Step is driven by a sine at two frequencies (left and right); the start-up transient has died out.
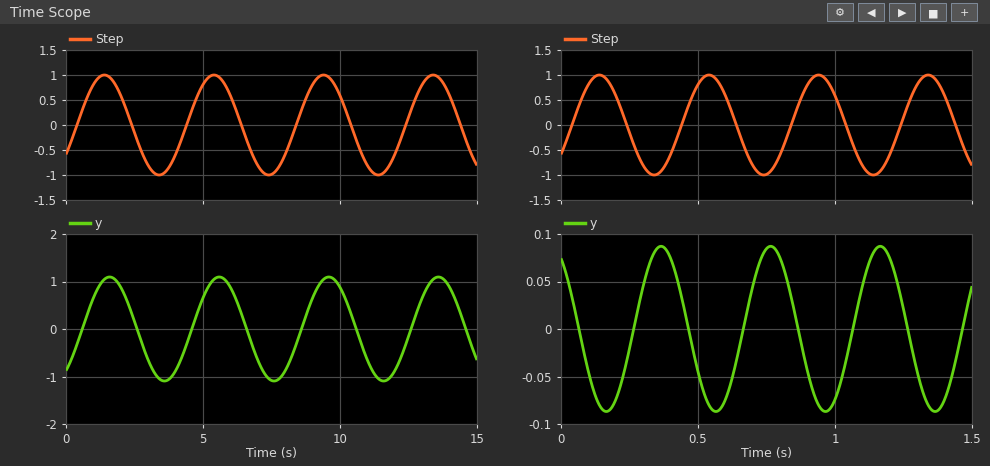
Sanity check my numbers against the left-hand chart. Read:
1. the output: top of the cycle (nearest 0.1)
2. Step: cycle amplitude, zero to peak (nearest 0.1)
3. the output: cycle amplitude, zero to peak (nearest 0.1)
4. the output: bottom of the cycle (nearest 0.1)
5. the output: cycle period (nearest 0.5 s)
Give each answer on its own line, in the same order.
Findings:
1.1
1.0
1.1
-1.1
4.0 s
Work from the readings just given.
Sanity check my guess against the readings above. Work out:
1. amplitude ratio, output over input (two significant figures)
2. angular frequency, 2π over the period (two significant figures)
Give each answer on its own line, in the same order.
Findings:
1.1
1.6 rad/s
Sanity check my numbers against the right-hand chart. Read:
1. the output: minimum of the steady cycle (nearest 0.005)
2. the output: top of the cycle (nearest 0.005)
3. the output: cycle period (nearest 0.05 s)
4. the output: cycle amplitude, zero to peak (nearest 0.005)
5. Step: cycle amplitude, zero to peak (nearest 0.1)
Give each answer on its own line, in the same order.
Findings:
-0.085
0.085
0.40 s
0.085
1.0
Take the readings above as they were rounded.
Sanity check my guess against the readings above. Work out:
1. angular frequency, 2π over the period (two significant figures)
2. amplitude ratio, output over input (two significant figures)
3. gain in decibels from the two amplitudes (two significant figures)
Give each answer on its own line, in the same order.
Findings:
16 rad/s
0.085
-21 dB
